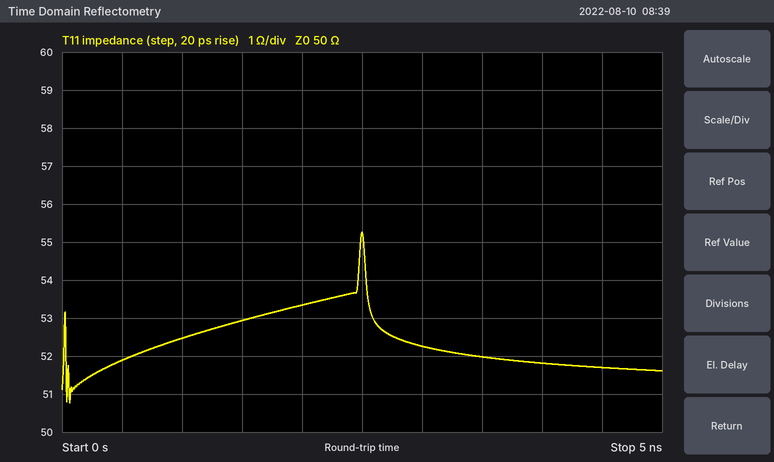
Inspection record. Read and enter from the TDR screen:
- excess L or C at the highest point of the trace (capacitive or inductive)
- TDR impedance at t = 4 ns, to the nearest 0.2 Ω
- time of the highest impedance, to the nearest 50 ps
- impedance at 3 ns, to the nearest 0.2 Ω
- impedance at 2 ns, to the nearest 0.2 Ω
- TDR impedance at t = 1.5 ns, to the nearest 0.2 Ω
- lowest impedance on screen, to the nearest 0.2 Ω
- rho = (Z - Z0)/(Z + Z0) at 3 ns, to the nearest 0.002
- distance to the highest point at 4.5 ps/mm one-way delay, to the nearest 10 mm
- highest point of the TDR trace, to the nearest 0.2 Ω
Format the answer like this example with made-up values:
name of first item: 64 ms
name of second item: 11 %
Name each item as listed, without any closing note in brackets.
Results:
excess L or C at the highest point of the trace: inductive
TDR impedance at t = 4 ns, to the nearest 0.2 Ω: 51.8 Ω
time of the highest impedance, to the nearest 50 ps: 2.50 ns
impedance at 3 ns, to the nearest 0.2 Ω: 52.2 Ω
impedance at 2 ns, to the nearest 0.2 Ω: 53.4 Ω
TDR impedance at t = 1.5 ns, to the nearest 0.2 Ω: 53.0 Ω
lowest impedance on screen, to the nearest 0.2 Ω: 50.8 Ω
rho = (Z - Z0)/(Z + Z0) at 3 ns, to the nearest 0.002: +0.022
distance to the highest point at 4.5 ps/mm one-way delay, to the nearest 10 mm: 280 mm
highest point of the TDR trace, to the nearest 0.2 Ω: 55.2 Ω
